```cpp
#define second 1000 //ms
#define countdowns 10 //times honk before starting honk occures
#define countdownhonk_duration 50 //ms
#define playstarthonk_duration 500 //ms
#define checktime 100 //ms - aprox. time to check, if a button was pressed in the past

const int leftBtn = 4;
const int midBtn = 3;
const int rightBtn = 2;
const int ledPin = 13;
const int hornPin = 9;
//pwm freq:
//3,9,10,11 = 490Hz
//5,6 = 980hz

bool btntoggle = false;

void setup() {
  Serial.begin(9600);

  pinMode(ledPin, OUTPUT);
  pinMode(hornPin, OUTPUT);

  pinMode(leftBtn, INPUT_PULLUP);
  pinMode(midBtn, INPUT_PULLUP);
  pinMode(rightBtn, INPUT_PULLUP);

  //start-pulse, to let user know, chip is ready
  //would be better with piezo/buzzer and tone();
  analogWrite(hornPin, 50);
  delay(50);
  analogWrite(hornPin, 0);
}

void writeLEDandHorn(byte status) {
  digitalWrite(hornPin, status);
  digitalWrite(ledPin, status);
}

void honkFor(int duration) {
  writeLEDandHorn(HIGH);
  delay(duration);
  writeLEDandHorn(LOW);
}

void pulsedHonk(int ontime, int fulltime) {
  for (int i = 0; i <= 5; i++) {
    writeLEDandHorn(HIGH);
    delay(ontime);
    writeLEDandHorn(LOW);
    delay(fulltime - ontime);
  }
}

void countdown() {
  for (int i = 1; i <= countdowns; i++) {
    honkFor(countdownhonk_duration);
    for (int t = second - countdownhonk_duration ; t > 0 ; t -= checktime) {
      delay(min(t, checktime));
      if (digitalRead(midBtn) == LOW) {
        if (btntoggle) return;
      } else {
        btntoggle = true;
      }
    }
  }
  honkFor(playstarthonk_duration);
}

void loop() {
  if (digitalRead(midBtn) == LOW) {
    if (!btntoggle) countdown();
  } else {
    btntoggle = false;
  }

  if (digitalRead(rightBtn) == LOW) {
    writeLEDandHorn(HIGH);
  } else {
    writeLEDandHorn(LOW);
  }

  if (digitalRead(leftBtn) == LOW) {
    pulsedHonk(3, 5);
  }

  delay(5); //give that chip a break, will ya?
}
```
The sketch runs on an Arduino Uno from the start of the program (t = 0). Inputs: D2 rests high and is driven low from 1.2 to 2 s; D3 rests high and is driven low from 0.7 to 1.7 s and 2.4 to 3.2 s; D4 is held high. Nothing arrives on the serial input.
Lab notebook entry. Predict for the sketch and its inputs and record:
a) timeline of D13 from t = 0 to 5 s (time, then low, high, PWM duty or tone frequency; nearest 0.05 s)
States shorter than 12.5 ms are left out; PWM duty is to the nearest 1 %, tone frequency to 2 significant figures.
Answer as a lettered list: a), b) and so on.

a) 0 s low; 0.7 s high; 0.75 s low; 1.7 s high; 1.75 s low
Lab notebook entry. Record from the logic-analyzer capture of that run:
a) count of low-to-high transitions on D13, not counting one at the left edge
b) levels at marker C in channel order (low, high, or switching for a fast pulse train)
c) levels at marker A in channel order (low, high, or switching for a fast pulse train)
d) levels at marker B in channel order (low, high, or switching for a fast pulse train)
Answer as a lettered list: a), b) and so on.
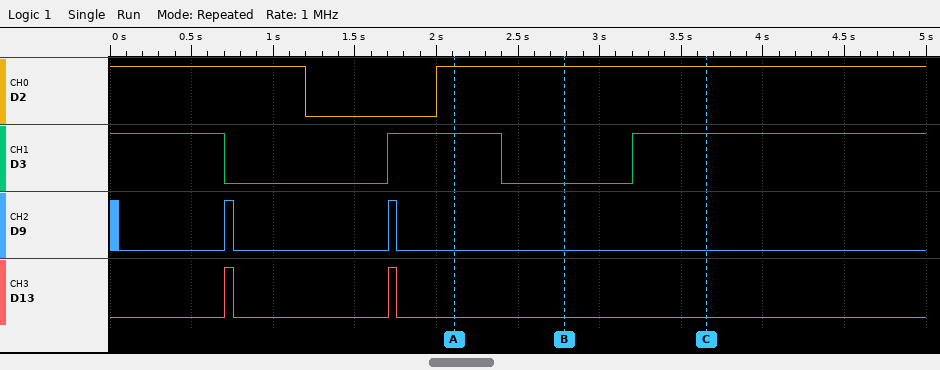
a) 2
b) D2 high, D3 high, D9 low, D13 low
c) D2 high, D3 high, D9 low, D13 low
d) D2 high, D3 low, D9 low, D13 low
